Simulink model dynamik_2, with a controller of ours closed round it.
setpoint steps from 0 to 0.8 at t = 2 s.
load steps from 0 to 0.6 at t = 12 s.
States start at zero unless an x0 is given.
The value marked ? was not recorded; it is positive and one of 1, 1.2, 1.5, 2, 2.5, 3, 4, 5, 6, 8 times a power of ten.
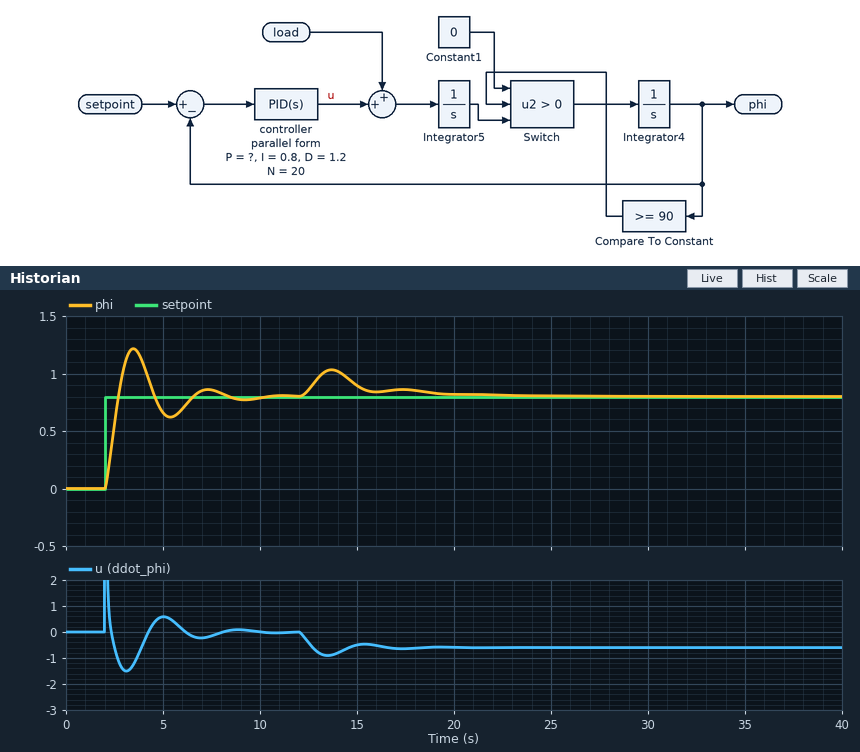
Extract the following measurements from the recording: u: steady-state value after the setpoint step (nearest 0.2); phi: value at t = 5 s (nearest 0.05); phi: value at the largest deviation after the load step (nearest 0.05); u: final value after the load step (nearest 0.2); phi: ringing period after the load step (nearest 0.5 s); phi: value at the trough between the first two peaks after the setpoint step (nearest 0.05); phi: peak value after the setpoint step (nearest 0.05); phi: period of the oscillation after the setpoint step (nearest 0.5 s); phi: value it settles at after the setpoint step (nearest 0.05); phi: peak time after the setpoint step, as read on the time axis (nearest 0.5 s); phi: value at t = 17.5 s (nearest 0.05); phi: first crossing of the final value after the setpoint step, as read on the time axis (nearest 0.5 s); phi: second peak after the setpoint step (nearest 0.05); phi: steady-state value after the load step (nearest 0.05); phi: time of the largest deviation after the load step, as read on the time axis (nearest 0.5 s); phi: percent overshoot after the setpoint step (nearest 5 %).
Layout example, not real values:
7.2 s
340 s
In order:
0.0
0.65
1.05
-0.6
3.5 s
0.60
1.20
4.0 s
0.80
3.5 s
0.85
2.5 s
0.85
0.80
13.5 s
50 %
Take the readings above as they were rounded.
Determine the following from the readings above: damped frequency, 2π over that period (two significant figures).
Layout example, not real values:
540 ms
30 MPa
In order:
1.6 rad/s
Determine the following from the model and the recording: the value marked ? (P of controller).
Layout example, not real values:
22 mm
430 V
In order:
3
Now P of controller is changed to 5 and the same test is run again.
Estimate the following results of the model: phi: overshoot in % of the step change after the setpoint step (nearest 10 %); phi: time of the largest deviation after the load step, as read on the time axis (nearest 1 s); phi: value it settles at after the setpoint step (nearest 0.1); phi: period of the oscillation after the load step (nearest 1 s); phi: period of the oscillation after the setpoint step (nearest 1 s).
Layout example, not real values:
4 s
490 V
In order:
60 %
13 s
0.8
3 s
3 s
